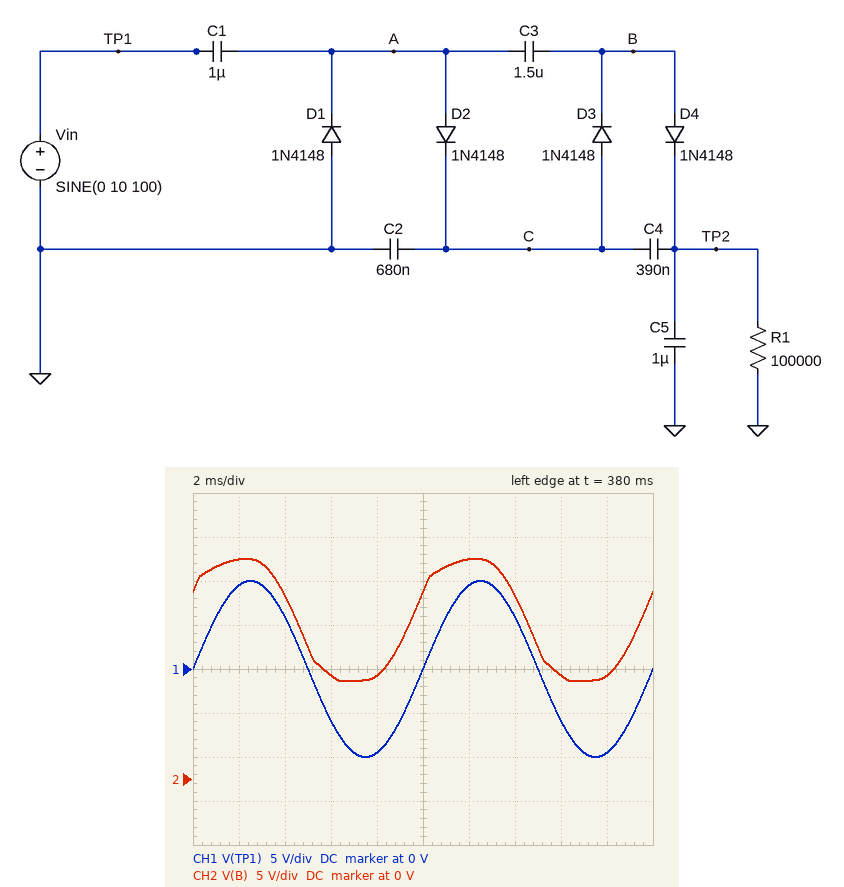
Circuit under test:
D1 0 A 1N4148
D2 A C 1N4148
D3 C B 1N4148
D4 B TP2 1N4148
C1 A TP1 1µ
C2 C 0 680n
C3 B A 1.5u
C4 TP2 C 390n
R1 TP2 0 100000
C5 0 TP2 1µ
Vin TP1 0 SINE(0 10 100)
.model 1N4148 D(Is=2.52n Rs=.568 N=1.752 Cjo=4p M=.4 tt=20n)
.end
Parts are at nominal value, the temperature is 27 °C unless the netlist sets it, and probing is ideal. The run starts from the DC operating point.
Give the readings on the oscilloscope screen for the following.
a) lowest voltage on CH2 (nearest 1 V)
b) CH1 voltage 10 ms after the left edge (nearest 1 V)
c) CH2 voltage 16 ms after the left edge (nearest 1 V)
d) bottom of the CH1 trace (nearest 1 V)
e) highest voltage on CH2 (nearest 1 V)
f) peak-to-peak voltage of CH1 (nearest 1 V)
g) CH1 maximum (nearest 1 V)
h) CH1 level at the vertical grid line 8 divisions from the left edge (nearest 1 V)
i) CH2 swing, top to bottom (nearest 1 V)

11 V
0 V
12 V
-10 V
25 V
20 V
10 V
-6 V
14 V
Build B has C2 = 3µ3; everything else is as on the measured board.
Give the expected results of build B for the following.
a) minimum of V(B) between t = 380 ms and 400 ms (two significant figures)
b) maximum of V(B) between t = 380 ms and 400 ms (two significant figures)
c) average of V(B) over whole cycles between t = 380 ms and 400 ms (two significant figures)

13 V
26 V
19 V
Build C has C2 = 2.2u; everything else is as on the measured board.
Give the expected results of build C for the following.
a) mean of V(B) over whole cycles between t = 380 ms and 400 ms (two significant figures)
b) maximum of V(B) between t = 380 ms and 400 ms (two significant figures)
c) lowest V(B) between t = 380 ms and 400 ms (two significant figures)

19 V
26 V
12 V
